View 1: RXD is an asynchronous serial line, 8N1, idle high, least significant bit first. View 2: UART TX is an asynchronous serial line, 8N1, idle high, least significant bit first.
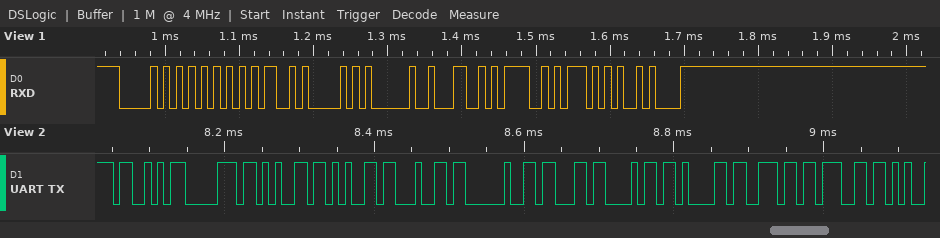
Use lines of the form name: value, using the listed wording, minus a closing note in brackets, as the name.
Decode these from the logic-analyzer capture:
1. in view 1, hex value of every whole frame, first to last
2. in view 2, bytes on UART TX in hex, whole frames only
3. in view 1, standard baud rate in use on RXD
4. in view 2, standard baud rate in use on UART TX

in view 1, hex value of every whole frame, first to last: 0x50 0x55 0x4D 0x50 0x20 0x4C 0x4F 0x57 0x0A
in view 2, bytes on UART TX in hex, whole frames only: 0x53 0x70 0x65 0x65 0x64 0x20 0x63 0x68 0x61 0x6E 0x67
in view 1, standard baud rate in use on RXD: 115200 baud
in view 2, standard baud rate in use on UART TX: 115200 baud
